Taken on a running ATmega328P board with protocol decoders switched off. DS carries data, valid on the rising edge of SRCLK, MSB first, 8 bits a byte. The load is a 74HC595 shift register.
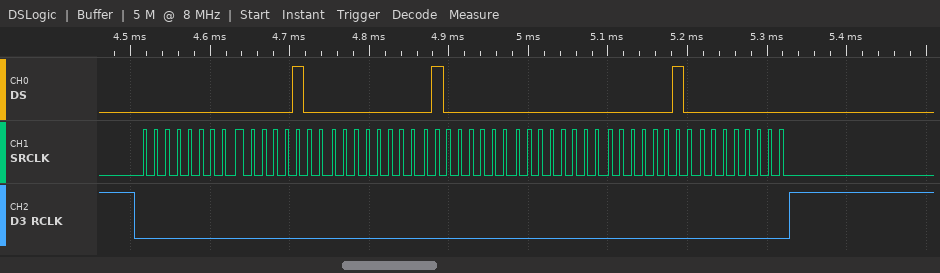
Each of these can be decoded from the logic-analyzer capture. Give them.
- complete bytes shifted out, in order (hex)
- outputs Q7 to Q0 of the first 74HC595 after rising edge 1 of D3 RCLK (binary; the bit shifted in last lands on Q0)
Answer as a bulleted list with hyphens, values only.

- 0x00 0x04 0x00 0x40 0x00 0x02 0x00
- 00000000
